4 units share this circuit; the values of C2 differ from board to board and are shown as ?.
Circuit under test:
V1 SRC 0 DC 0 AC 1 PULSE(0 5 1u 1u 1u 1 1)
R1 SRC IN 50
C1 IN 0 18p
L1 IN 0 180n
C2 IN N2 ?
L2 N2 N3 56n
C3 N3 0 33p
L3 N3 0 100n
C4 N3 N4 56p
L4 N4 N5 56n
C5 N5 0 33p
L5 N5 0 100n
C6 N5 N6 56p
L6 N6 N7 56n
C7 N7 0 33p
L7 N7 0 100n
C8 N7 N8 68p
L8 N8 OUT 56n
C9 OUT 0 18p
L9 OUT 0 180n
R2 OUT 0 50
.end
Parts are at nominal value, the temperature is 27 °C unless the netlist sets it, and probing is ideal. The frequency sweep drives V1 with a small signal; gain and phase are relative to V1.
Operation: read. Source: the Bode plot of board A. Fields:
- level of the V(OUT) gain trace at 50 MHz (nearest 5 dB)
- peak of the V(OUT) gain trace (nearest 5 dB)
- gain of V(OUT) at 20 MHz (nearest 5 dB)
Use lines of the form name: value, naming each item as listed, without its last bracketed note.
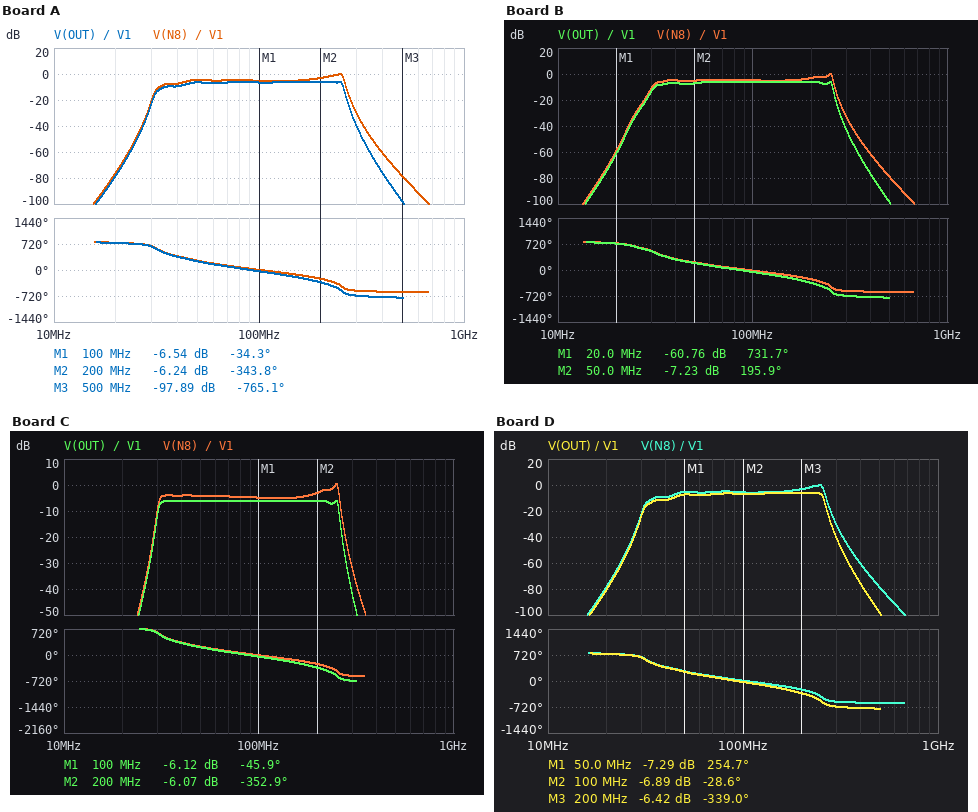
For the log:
level of the V(OUT) gain trace at 50 MHz: -5 dB
peak of the V(OUT) gain trace: -5 dB
gain of V(OUT) at 20 MHz: -80 dB
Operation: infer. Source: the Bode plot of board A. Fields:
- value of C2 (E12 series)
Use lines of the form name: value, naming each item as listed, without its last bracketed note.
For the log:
value of C2: 33 pF
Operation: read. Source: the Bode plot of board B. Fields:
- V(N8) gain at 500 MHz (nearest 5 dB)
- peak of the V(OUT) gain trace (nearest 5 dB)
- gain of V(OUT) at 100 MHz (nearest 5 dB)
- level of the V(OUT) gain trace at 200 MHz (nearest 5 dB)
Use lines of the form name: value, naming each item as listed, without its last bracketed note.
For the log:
V(N8) gain at 500 MHz: -80 dB
peak of the V(OUT) gain trace: -5 dB
gain of V(OUT) at 100 MHz: -5 dB
level of the V(OUT) gain trace at 200 MHz: -5 dB
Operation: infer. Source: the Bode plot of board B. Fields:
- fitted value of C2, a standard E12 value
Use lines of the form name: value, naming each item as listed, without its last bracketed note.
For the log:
fitted value of C2, a standard E12 value: 120 pF
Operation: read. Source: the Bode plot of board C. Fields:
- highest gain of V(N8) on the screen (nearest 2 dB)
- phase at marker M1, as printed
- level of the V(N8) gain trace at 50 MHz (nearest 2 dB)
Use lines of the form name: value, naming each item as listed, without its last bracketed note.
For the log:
highest gain of V(N8) on the screen: 0 dB
phase at marker M1, as printed: -45.9 deg
level of the V(N8) gain trace at 50 MHz: -4 dB
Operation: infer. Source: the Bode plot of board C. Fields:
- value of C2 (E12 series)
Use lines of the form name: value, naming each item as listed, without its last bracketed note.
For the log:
value of C2: 56 pF
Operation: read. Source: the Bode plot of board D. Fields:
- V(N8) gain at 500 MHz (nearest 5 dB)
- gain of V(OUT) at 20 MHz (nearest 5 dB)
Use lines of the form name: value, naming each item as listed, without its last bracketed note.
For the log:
V(N8) gain at 500 MHz: -80 dB
gain of V(OUT) at 20 MHz: -80 dB
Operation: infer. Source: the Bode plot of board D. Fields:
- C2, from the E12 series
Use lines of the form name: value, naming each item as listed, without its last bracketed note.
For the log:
C2, from the E12 series: 27 pF
